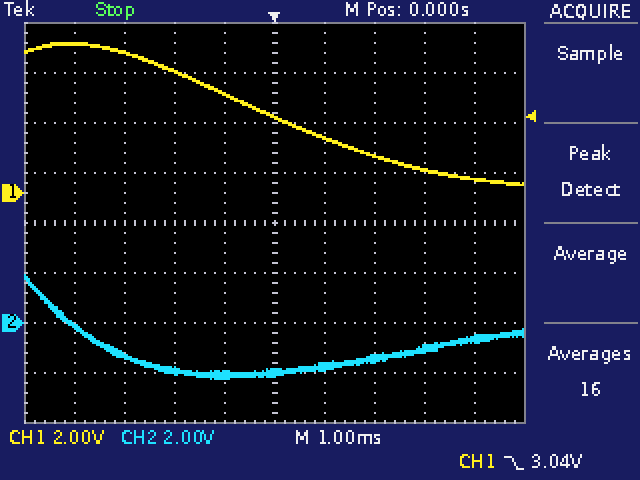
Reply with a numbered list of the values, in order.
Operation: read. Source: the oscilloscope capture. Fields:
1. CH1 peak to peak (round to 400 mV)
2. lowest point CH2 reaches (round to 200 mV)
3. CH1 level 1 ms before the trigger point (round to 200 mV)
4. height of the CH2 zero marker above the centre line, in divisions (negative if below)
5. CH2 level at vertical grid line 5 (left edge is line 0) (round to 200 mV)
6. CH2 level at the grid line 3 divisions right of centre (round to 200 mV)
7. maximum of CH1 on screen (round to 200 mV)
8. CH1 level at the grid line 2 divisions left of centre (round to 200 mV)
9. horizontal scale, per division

1. 5.6 V
2. -2.2 V
3. 4.0 V
4. -2.0 div
5. -2.0 V
6. -1.0 V
7. 6.0 V
8. 4.8 V
9. 1 ms
